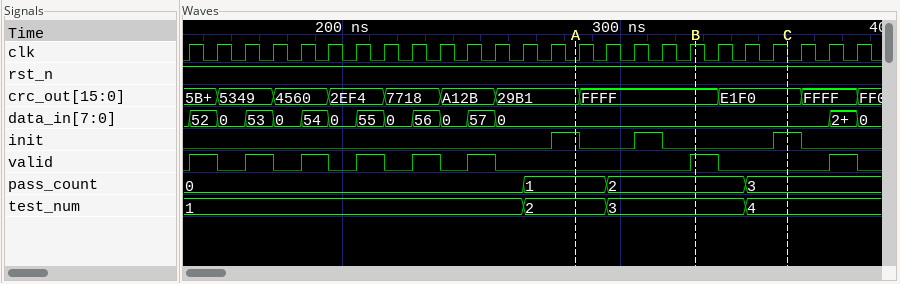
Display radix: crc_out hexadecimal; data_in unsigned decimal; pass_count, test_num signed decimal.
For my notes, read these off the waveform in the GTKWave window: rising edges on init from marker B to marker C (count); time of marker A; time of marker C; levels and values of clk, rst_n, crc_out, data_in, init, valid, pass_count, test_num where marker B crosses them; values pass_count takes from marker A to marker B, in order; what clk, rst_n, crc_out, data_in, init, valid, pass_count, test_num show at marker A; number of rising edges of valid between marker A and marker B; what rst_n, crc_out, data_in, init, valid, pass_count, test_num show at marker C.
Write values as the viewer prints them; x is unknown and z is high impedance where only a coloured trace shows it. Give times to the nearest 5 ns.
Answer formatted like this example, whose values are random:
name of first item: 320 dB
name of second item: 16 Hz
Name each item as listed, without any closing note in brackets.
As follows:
rising edges on init from marker B to marker C: 1
time of marker A: 285 ns
time of marker C: 360 ns
levels and values of clk, rst_n, crc_out, data_in, init, valid, pass_count, test_num where marker B crosses them: clk=1, rst_n=1, crc_out=FFFF, data_in=0, init=0, valid=1, pass_count=2, test_num=3
values pass_count takes from marker A to marker B, in order: 1, 2
what clk, rst_n, crc_out, data_in, init, valid, pass_count, test_num show at marker A: clk=0, rst_n=1, crc_out=29B1, data_in=0, init=1, valid=0, pass_count=1, test_num=2
number of rising edges of valid between marker A and marker B: 1
what rst_n, crc_out, data_in, init, valid, pass_count, test_num show at marker C: rst_n=1, crc_out=E1F0, data_in=0, init=1, valid=0, pass_count=3, test_num=4
